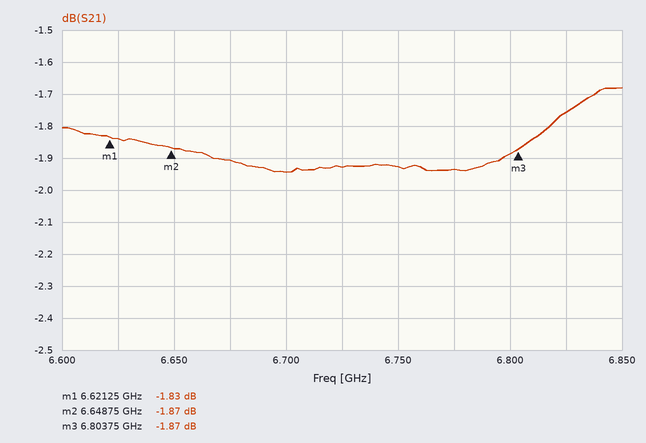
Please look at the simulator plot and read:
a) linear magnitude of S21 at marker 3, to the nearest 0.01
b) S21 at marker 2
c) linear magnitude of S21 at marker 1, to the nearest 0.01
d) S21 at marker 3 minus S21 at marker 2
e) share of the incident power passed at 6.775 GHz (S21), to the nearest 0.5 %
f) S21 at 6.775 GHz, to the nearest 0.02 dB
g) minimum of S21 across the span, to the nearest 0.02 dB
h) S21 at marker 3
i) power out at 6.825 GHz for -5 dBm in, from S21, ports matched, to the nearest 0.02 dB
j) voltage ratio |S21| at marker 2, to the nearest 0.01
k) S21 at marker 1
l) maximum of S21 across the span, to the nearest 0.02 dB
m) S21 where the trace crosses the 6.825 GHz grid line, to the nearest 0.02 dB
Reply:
0.81
-1.87 dB
0.81
0.00 dB
64.0 %
-1.94 dB
-1.94 dB
-1.87 dB
-6.76 dBm
0.81
-1.83 dB
-1.68 dB
-1.76 dB
